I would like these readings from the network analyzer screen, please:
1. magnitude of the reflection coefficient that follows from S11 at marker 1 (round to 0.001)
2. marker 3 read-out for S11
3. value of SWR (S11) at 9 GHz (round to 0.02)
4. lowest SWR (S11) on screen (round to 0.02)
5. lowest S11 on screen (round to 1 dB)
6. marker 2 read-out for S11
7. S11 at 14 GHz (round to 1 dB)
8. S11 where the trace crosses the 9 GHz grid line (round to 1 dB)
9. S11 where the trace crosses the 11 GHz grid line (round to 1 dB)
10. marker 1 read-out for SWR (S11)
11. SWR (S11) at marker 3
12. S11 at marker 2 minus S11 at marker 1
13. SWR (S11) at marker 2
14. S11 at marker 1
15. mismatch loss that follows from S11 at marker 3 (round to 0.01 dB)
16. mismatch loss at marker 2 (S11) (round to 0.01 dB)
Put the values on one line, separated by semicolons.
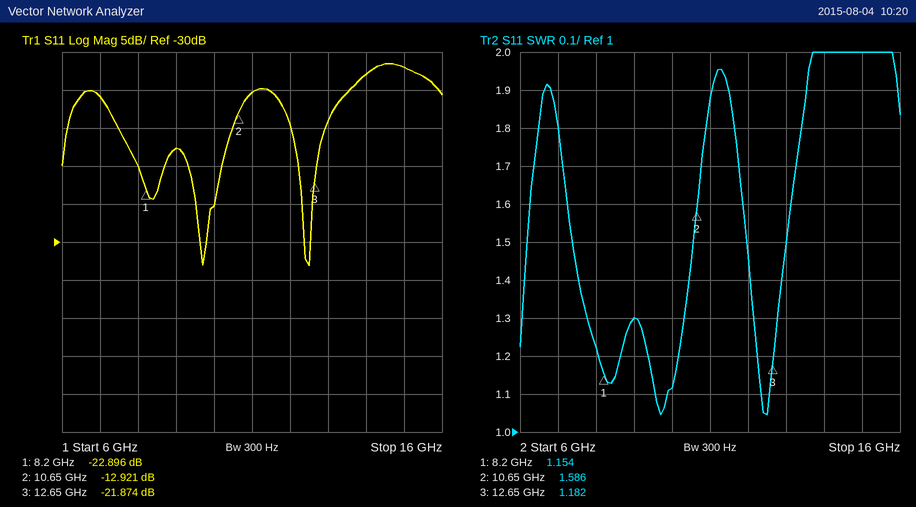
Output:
0.072; -21.874 dB; 1.30; 1.04; -33 dB; -12.921 dB; -8 dB; -18 dB; -10 dB; 1.154; 1.182; 9.975 dB; 1.586; -22.896 dB; 0.03 dB; 0.23 dB
